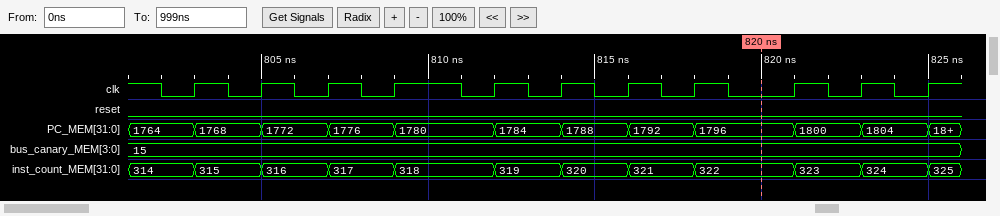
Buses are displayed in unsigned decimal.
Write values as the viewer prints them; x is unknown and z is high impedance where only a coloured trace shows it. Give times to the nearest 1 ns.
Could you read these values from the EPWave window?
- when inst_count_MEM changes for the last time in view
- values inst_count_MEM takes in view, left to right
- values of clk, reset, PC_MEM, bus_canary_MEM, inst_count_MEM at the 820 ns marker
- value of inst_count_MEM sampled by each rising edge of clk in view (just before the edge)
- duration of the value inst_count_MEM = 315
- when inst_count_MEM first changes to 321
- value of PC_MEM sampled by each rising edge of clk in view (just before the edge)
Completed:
825 ns
314, 315, 316, 317, 318, 319, 320, 321, 322, 323, 324, 325
clk=0, reset=0, PC_MEM=1796, bus_canary_MEM=15, inst_count_MEM=322
314, 315, 316, 317, 318, 319, 320, 321, 322, 323, 324
2 ns
816 ns
1764, 1768, 1772, 1776, 1780, 1784, 1788, 1792, 1796, 1800, 1804
